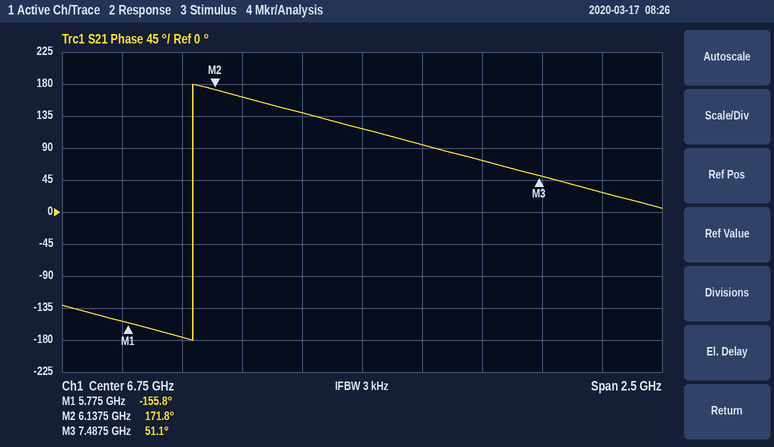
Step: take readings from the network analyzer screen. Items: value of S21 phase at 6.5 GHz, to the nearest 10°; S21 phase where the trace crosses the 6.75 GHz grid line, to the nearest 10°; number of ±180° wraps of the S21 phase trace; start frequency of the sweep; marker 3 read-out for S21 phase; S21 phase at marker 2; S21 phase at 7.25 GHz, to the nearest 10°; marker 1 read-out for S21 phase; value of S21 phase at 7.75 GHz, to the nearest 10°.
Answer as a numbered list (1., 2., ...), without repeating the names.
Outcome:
1. 140°
2. 120°
3. 1
4. 5.5 GHz
5. 51.1°
6. 171.8°
7. 70°
8. -155.8°
9. 30°
